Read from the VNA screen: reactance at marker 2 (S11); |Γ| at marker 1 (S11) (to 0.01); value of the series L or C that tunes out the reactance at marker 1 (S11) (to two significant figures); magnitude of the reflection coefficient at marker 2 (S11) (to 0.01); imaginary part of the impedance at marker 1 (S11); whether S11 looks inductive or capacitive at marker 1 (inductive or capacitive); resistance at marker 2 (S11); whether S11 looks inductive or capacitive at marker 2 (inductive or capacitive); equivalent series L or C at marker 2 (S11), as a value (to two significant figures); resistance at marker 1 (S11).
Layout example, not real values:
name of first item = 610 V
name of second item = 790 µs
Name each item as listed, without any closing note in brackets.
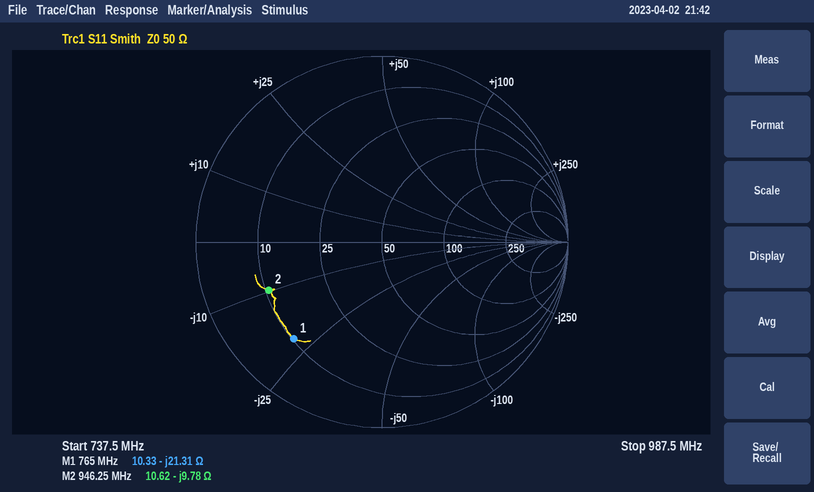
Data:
reactance at marker 2 = -9.78 Ω
|Γ| at marker 1 (S11) = 0.70
value of the series L or C that tunes out the reactance at marker 1 (S11) = 4.4 nH
magnitude of the reflection coefficient at marker 2 (S11) = 0.66
imaginary part of the impedance at marker 1 = -21.31 Ω
whether S11 looks inductive or capacitive at marker 1 = capacitive
resistance at marker 2 = 10.62 Ω
whether S11 looks inductive or capacitive at marker 2 = capacitive
equivalent series L or C at marker 2 (S11), as a value = 17 pF
resistance at marker 1 = 10.33 Ω
